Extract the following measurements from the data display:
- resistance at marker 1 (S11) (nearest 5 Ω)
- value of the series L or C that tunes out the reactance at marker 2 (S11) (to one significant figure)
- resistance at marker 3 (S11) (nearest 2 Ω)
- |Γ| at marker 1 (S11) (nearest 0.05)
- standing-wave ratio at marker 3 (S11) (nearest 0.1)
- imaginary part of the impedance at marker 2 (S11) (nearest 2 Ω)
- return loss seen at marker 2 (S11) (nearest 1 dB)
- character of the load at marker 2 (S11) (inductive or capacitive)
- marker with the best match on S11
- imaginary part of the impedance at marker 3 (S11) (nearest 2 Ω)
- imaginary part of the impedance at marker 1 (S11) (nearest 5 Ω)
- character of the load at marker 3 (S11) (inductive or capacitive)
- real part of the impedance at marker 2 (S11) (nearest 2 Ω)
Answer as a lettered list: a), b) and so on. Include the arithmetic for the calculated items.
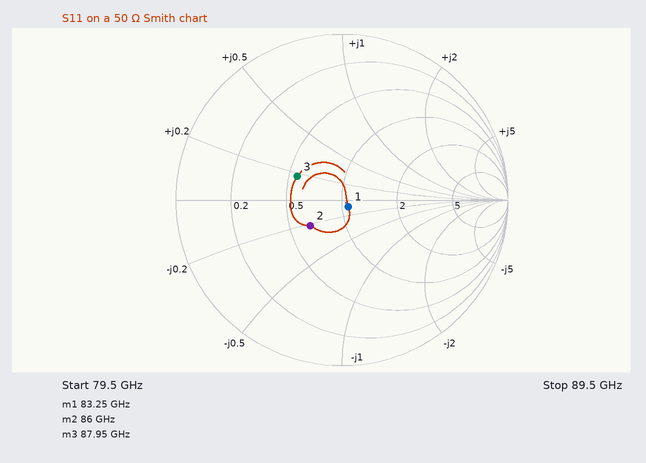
a) 55 Ω
b) L = 10 Ω/(2π × 86 GHz) ≈ 18.5 pH, so 20 pH to one significant figure
c) 28 Ω
d) 0.05
e) 1.9
f) -10 Ω
g) 12 dB
h) capacitive
i) marker 1
j) +8 Ω
k) -5 Ω
l) inductive
m) 32 Ω
